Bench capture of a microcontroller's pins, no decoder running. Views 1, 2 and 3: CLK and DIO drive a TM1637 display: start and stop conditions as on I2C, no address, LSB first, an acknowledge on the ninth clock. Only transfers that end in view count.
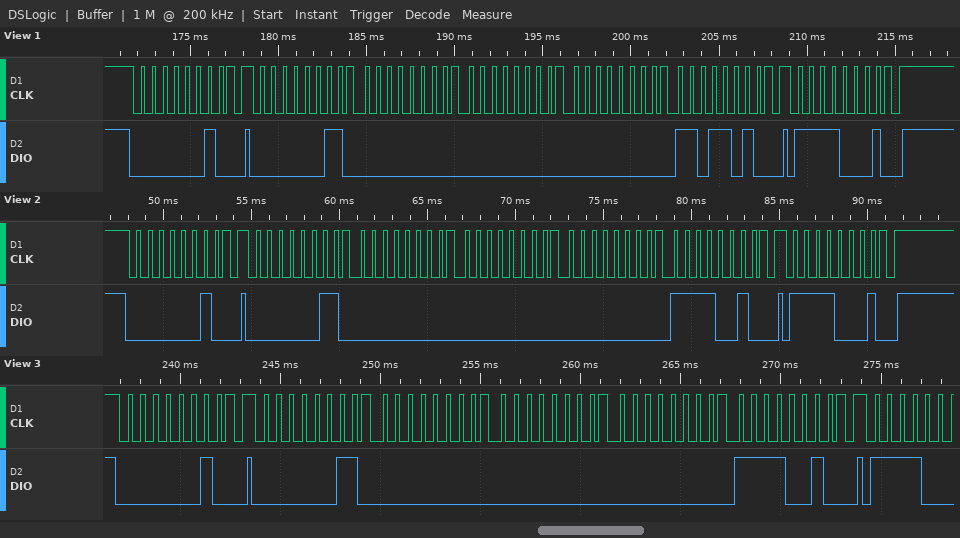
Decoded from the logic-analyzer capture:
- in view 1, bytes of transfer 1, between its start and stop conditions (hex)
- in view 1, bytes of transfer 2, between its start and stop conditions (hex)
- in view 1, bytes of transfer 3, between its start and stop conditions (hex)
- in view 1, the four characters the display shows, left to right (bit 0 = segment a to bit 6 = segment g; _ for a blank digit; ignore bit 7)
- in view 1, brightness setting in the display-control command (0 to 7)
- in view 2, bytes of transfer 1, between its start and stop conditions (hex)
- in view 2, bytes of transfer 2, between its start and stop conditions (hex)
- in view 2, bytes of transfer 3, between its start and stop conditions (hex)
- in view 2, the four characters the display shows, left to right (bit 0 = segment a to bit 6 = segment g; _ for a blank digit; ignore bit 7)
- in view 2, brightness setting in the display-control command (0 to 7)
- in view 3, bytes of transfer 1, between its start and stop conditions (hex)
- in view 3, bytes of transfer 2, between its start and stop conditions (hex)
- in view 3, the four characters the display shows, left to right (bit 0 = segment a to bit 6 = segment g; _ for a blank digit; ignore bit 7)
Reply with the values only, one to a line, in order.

40
C0 00 00 00 5B
8F
___2
7
40
C0 00 00 00 4F
8F
___3
7
40
C0 00 00 00 4F
___3
